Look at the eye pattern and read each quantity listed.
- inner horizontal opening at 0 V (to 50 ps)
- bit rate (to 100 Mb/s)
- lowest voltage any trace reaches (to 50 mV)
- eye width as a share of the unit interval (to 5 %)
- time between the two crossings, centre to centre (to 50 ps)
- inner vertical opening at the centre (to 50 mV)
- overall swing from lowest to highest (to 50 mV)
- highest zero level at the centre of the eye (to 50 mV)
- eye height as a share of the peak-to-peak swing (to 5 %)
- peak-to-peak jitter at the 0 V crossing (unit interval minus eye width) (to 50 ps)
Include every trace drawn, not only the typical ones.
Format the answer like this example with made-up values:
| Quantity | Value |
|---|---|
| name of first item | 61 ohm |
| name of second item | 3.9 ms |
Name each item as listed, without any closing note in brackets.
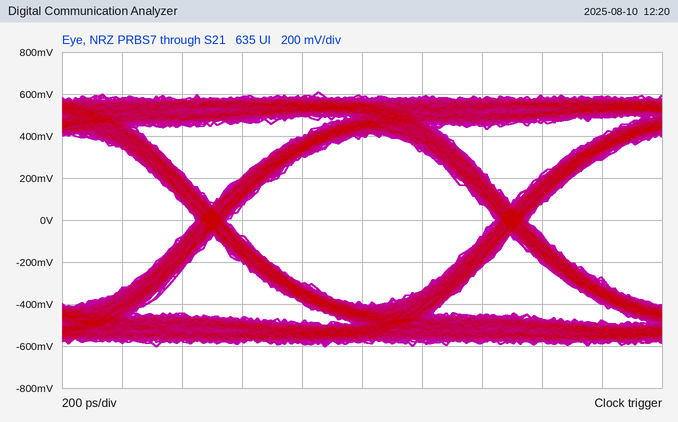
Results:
| Quantity | Value |
|---|---|
| inner horizontal opening at 0 V | 900 ps |
| bit rate | 1.0 Gb/s |
| lowest voltage any trace reaches | -600 mV |
| eye width as a share of the unit interval | 90 % |
| time between the two crossings, centre to centre | 1.00 ns |
| inner vertical opening at the centre | 800 mV |
| overall swing from lowest to highest | 1.20 V |
| highest zero level at the centre of the eye | -400 mV |
| eye height as a share of the peak-to-peak swing | 65 % |
| peak-to-peak jitter at the 0 V crossing (unit interval minus eye width) | 100 ps |
